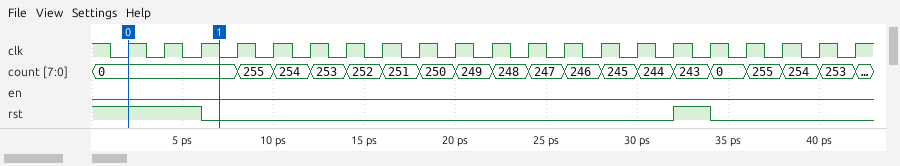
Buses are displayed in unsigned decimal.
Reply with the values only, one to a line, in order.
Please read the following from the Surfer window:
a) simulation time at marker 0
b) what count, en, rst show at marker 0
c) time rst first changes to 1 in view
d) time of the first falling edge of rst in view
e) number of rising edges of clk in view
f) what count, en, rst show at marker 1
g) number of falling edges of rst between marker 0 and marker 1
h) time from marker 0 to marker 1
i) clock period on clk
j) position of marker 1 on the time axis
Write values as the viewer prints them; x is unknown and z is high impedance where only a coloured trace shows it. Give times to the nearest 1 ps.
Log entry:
2 ps
count=0, en=0, rst=1
32 ps
6 ps
21
count=0, en=0, rst=0
1
5 ps
2 ps
7 ps
